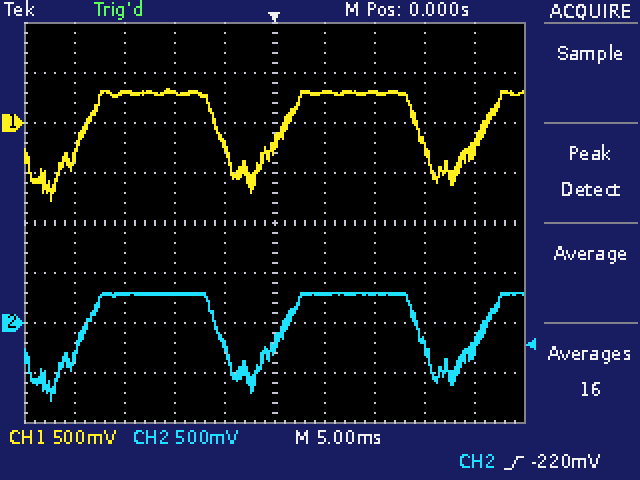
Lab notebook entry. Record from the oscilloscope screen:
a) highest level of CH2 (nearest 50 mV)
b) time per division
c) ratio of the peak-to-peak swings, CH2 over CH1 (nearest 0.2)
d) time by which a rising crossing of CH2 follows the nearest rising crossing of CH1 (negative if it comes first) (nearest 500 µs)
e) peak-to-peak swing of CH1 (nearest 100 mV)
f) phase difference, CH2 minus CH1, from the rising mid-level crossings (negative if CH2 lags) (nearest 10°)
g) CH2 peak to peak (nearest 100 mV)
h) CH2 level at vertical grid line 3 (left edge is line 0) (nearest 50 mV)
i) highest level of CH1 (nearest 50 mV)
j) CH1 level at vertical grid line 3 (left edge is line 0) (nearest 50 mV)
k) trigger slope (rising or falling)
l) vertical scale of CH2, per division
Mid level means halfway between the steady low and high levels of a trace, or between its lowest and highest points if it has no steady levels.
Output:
300 mV
5 ms
1.0
0.0 ms
1.10 V
0°
1.10 V
300 mV
350 mV
300 mV
rising
500 mV
